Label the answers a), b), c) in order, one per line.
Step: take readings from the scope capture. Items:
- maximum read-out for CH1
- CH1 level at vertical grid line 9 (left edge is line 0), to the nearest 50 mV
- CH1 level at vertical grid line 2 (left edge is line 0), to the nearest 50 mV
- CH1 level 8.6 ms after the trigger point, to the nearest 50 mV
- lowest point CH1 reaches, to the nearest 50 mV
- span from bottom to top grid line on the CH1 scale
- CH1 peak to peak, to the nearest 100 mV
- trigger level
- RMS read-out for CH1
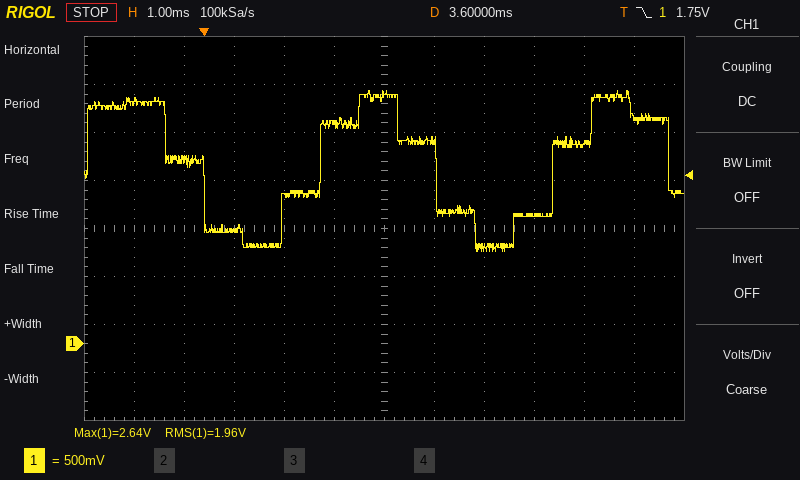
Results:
a) 2.64 V
b) 1.35 V
c) 1.90 V
d) 2.35 V
e) 950 mV
f) 4 V
g) 1.70 V
h) 1.75 V
i) 1.96 V
